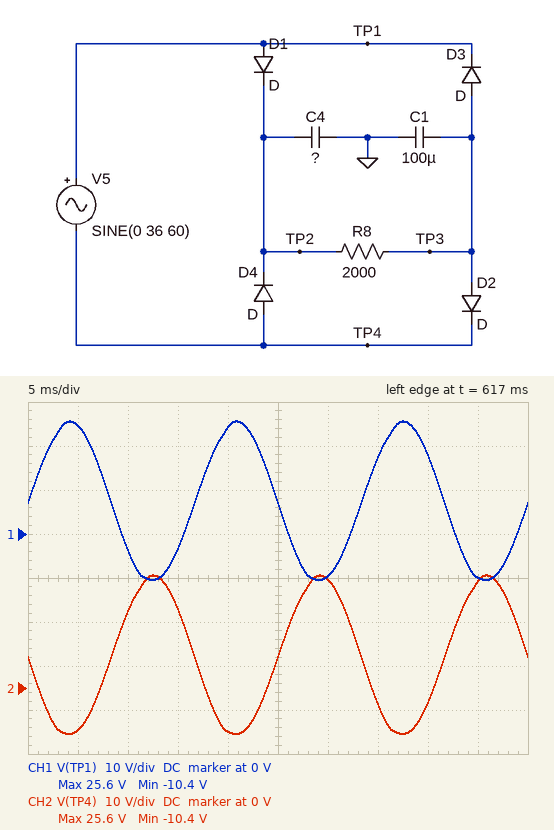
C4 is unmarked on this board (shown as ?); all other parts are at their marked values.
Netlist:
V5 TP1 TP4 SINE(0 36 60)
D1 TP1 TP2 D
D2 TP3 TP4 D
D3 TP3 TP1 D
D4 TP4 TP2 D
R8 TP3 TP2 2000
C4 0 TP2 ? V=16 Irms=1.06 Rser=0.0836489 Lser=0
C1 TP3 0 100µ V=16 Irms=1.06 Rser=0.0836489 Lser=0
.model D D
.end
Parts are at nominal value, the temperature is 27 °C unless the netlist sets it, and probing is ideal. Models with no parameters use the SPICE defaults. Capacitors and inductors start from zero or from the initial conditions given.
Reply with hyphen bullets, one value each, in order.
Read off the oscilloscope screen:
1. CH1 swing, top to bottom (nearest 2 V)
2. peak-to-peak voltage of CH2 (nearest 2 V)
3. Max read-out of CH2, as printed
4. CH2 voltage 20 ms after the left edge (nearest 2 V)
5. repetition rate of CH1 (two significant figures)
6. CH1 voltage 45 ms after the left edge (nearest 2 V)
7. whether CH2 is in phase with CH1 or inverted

- 36 V
- 36 V
- 25.6 V
- -10 V
- 60 Hz
- -10 V
- inverted
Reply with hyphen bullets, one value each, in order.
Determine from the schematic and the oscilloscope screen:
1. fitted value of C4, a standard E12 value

- 39 µF
